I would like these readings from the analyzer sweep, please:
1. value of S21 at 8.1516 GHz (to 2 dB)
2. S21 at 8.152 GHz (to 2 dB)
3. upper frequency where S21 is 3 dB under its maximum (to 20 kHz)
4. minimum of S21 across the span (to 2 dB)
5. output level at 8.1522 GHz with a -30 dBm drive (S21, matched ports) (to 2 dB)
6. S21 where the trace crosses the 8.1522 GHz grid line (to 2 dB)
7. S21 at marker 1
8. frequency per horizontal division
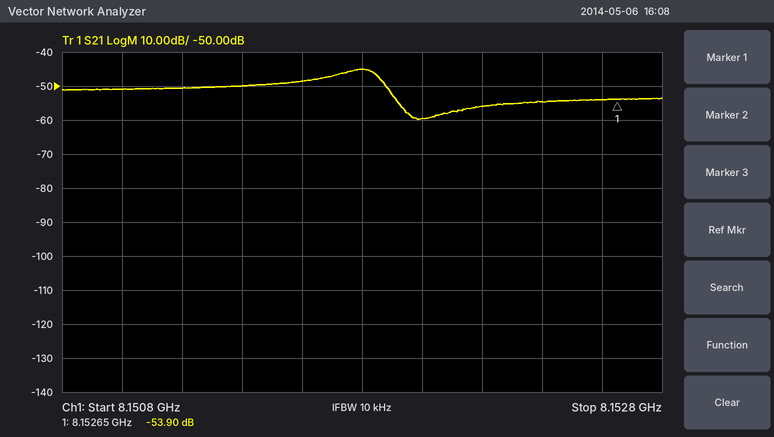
-48 dB
-60 dB
8.15186 GHz
-60 dB
-86 dBm
-56 dB
-53.90 dB
200 kHz
